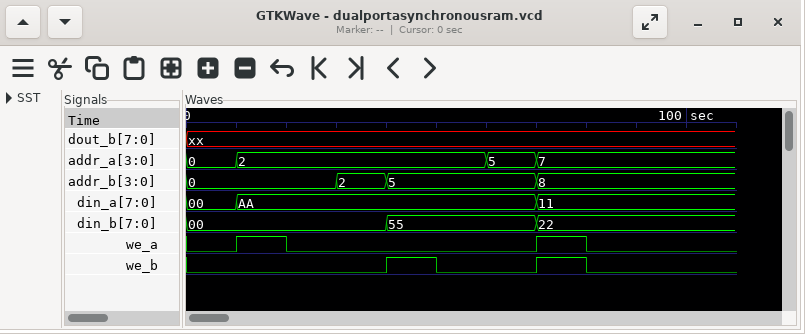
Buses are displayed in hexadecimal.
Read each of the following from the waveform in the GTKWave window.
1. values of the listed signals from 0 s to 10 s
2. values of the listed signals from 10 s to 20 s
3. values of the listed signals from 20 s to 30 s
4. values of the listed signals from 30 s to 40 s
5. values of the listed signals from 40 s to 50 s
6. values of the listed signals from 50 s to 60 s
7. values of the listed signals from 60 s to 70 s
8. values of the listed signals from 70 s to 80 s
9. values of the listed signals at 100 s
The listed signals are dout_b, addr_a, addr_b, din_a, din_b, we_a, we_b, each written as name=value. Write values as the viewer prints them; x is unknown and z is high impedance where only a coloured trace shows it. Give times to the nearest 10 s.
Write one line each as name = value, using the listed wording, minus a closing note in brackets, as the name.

values of the listed signals from 0 s to 10 s = dout_b=xx, addr_a=0, addr_b=0, din_a=00, din_b=00, we_a=0, we_b=0
values of the listed signals from 10 s to 20 s = dout_b=xx, addr_a=2, addr_b=0, din_a=AA, din_b=00, we_a=1, we_b=0
values of the listed signals from 20 s to 30 s = dout_b=xx, addr_a=2, addr_b=0, din_a=AA, din_b=00, we_a=0, we_b=0
values of the listed signals from 30 s to 40 s = dout_b=xx, addr_a=2, addr_b=2, din_a=AA, din_b=00, we_a=0, we_b=0
values of the listed signals from 40 s to 50 s = dout_b=xx, addr_a=2, addr_b=5, din_a=AA, din_b=55, we_a=0, we_b=1
values of the listed signals from 50 s to 60 s = dout_b=xx, addr_a=2, addr_b=5, din_a=AA, din_b=55, we_a=0, we_b=0
values of the listed signals from 60 s to 70 s = dout_b=xx, addr_a=5, addr_b=5, din_a=AA, din_b=55, we_a=0, we_b=0
values of the listed signals from 70 s to 80 s = dout_b=xx, addr_a=7, addr_b=8, din_a=11, din_b=22, we_a=1, we_b=1
values of the listed signals at 100 s = dout_b=xx, addr_a=7, addr_b=8, din_a=11, din_b=22, we_a=0, we_b=0
